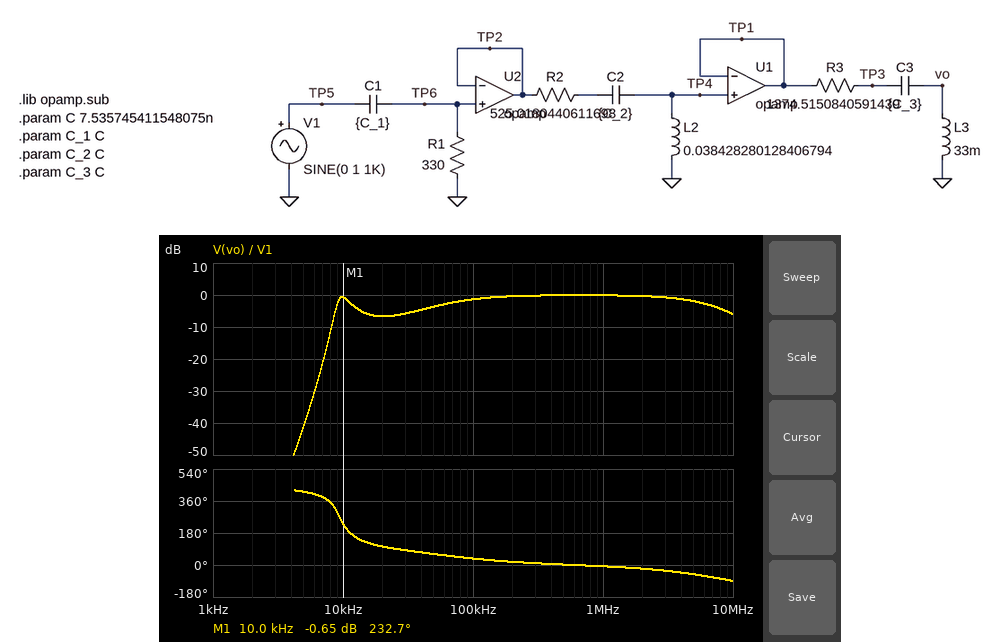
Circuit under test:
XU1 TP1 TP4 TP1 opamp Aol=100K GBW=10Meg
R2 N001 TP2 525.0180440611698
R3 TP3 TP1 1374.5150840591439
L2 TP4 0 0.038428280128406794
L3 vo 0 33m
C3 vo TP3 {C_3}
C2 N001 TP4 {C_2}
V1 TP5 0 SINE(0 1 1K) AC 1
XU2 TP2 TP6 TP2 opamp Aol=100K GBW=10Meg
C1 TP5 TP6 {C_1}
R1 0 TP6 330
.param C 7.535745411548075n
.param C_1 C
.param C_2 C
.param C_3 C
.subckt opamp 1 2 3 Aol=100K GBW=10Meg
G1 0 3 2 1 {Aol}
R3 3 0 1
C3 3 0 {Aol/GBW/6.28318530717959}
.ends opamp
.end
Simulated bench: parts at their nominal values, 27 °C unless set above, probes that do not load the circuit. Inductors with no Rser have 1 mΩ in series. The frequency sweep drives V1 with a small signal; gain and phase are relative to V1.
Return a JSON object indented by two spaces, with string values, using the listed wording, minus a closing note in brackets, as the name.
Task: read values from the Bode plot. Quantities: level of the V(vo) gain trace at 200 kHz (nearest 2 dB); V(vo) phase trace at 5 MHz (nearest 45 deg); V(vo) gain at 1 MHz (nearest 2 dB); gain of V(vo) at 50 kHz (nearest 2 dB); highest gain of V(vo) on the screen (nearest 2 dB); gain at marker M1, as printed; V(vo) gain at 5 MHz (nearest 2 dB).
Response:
{
  "level of the V(vo) gain trace at 200 kHz": "0 dB",
  "V(vo) phase trace at 5 MHz": "-45 deg",
  "V(vo) gain at 1 MHz": "0 dB",
  "gain of V(vo) at 50 kHz": "-4 dB",
  "highest gain of V(vo) on the screen": "0 dB",
  "gain at marker M1, as printed": "-0.65 dB",
  "V(vo) gain at 5 MHz": "-2 dB"
}
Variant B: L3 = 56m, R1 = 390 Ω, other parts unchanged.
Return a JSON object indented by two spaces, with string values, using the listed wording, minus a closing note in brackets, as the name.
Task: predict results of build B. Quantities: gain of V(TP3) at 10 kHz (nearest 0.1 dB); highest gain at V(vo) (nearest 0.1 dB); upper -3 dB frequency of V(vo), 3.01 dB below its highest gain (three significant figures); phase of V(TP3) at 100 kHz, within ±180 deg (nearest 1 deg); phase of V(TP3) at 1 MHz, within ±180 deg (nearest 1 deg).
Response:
{
  "gain of V(TP3) at 10 kHz": "-5.7 dB",
  "highest gain at V(vo)": "3.0 dB",
  "upper -3 dB frequency of V(vo), 3.01 dB below its highest gain": "10.8 kHz",
  "phase of V(TP3) at 100 kHz, within ±180 deg": "31 deg",
  "phase of V(TP3) at 1 MHz, within ±180 deg": "-8 deg"
}
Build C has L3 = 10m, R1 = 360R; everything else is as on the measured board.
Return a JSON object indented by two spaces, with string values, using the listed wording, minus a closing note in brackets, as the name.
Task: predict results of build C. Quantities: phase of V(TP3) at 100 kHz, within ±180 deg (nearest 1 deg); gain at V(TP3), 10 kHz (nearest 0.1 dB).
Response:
{
  "phase of V(TP3) at 100 kHz, within ±180 deg": "43 deg",
  "gain at V(TP3), 10 kHz": "-6.2 dB"
}
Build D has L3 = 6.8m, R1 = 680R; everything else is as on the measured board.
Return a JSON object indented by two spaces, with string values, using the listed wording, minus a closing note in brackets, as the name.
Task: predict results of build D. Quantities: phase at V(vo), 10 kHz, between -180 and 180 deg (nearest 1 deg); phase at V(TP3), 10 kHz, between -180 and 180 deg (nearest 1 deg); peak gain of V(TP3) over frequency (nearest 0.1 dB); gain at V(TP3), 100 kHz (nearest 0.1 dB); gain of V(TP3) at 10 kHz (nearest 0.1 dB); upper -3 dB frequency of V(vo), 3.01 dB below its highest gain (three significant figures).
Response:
{
  "phase at V(vo), 10 kHz, between -180 and 180 deg": "-87 deg",
  "phase at V(TP3), 10 kHz, between -180 and 180 deg": "93 deg",
  "peak gain of V(TP3) over frequency": "0.1 dB",
  "gain at V(TP3), 100 kHz": "-0.8 dB",
  "gain of V(TP3) at 10 kHz": "-0.5 dB",
  "upper -3 dB frequency of V(vo), 3.01 dB below its highest gain": "6.48 MHz"
}
